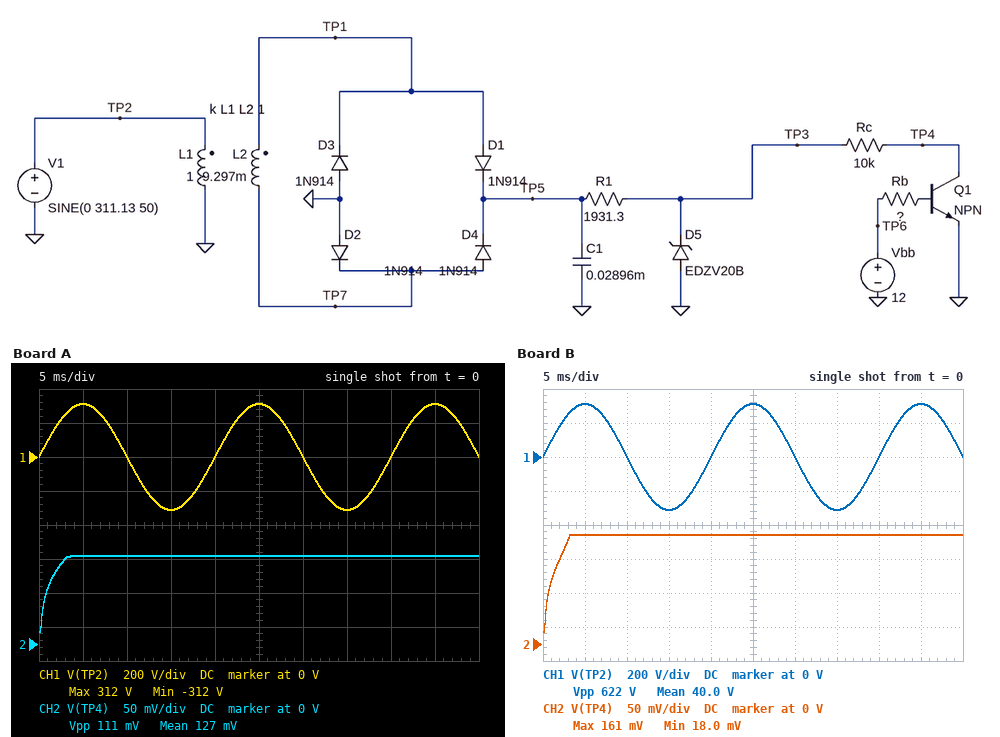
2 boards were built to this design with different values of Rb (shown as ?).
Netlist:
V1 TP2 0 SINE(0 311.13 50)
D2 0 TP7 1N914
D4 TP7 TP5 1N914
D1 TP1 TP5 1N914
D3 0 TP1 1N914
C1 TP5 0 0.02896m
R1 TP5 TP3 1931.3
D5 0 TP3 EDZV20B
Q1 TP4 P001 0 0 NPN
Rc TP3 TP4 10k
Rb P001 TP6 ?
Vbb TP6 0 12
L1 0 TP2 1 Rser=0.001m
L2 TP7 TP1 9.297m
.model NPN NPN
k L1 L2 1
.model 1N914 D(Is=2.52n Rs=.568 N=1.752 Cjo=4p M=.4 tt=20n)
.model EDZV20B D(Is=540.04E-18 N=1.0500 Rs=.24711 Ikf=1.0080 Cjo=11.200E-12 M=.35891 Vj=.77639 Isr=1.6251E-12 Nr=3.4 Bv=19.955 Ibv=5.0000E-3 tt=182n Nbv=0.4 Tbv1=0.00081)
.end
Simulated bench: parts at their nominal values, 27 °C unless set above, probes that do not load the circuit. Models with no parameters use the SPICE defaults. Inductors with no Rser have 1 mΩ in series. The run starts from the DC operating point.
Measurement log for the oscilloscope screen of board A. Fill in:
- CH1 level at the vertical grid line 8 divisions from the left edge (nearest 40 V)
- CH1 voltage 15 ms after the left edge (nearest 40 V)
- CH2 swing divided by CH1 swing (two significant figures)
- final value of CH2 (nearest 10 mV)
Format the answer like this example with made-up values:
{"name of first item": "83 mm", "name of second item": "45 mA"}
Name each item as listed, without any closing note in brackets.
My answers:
{"CH1 level at the vertical grid line 8 divisions from the left edge": "0 V", "CH1 voltage 15 ms after the left edge": "-320 V", "CH2 swing divided by CH1 swing": "0.00018", "final value of CH2": "130 mV"}
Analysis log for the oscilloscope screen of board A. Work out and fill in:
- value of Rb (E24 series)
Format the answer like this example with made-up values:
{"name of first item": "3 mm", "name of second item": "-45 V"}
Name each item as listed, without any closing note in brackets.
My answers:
{"value of Rb": "330 kΩ"}
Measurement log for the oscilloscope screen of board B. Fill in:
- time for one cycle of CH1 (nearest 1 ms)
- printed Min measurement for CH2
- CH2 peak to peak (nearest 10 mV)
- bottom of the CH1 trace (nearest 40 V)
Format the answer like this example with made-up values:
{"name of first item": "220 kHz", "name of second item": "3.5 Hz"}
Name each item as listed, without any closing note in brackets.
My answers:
{"time for one cycle of CH1": "20 ms", "printed Min measurement for CH2": "18.0 mV", "CH2 peak to peak": "140 mV", "bottom of the CH1 trace": "-320 V"}
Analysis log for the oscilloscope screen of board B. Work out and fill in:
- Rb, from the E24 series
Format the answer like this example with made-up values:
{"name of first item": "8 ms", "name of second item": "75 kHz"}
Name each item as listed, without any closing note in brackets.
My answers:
{"Rb, from the E24 series": "470 kΩ"}
